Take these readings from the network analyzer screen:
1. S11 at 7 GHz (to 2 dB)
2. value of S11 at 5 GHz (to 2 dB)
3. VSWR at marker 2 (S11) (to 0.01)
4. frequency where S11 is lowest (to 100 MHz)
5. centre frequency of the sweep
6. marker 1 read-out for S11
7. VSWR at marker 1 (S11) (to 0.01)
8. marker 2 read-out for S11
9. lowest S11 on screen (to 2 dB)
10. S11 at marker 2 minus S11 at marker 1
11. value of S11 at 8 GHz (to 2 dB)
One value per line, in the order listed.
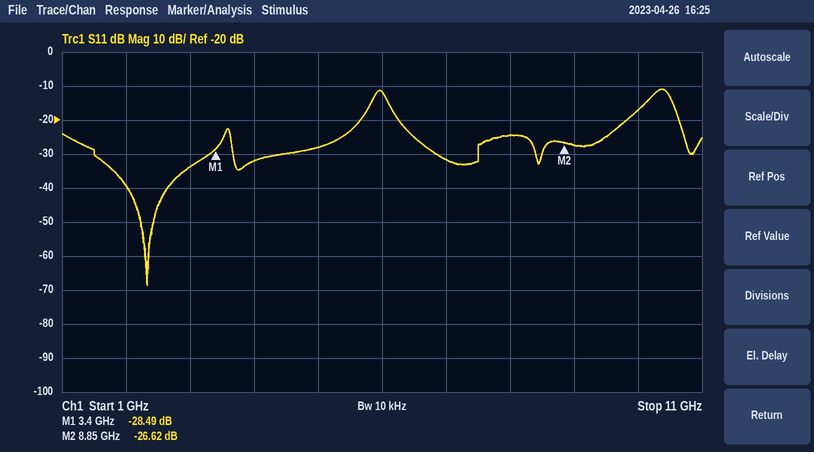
-32 dB
-28 dB
1.10
2.3 GHz
6 GHz
-28.49 dB
1.08
-26.62 dB
-68 dB
1.87 dB
-24 dB
